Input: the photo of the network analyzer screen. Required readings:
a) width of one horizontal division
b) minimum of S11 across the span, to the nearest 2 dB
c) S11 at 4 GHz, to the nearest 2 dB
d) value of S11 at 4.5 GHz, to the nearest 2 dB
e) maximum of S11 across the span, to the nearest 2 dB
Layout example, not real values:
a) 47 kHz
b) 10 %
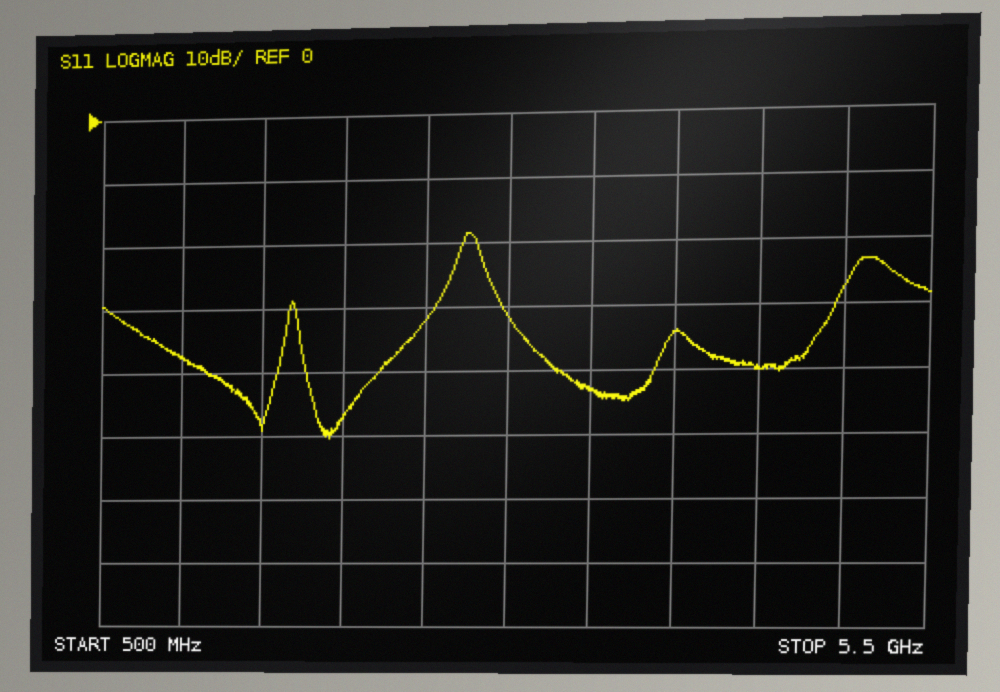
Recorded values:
a) 500 MHz
b) -50 dB
c) -34 dB
d) -40 dB
e) -18 dB
